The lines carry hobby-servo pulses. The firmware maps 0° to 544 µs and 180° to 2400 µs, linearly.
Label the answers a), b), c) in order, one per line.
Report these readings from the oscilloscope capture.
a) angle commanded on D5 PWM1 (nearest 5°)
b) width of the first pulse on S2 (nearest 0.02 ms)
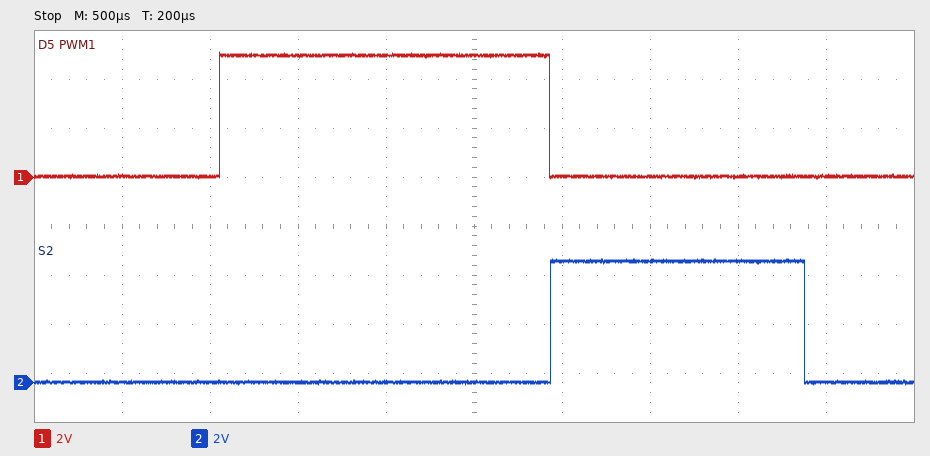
a) 130°
b) 1.44 ms
